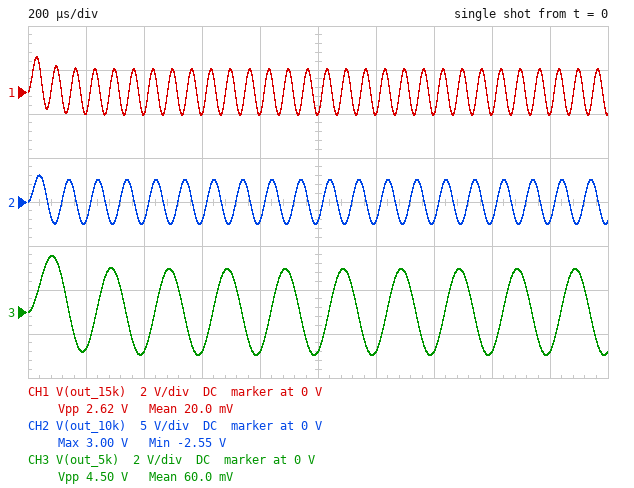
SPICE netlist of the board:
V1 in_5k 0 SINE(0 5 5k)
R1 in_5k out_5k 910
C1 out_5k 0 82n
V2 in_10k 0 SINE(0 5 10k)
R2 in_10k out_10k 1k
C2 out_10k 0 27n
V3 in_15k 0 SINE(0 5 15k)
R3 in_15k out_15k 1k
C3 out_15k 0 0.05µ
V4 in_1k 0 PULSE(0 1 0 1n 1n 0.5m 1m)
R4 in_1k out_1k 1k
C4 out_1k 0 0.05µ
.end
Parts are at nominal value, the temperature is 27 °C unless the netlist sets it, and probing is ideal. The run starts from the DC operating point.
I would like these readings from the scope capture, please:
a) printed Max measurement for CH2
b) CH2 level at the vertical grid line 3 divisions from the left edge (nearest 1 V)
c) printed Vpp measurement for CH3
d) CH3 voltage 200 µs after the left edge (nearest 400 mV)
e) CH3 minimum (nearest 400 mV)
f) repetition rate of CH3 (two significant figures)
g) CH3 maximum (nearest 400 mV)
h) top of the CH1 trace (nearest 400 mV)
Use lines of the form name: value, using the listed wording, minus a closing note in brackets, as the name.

printed Max measurement for CH2: 3.00 V
CH2 level at the vertical grid line 3 divisions from the left edge: -2 V
printed Vpp measurement for CH3: 4.50 V
CH3 voltage 200 µs after the left edge: -1.6 V
CH3 minimum: -2.0 V
repetition rate of CH3: 5.0 kHz
CH3 maximum: 2.4 V
top of the CH1 trace: 1.6 V
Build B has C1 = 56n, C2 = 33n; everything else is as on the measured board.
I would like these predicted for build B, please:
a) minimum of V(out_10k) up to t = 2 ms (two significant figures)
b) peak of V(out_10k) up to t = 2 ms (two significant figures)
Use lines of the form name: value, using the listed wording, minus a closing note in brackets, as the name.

minimum of V(out_10k) up to t = 2 ms: -2.2 V
peak of V(out_10k) up to t = 2 ms: 2.7 V
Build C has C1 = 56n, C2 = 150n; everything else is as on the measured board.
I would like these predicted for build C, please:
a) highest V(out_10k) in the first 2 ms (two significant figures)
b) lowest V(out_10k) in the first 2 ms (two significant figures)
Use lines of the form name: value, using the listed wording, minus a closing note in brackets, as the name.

highest V(out_10k) in the first 2 ms: 910 mV
lowest V(out_10k) in the first 2 ms: -530 mV
